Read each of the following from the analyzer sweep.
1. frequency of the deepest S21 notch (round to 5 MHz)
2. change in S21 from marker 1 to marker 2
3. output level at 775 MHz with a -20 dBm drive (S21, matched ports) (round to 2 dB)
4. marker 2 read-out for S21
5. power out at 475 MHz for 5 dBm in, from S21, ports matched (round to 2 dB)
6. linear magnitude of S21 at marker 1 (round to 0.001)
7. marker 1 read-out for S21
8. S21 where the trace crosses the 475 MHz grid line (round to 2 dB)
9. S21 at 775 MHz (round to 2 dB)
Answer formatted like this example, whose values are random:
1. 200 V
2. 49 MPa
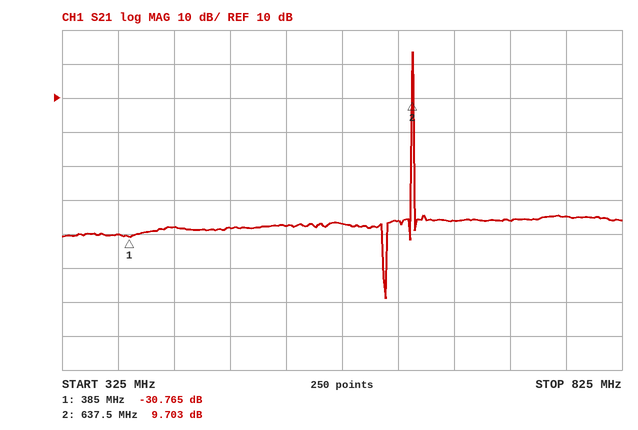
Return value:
1. 615 MHz
2. 40.468 dB
3. -44 dBm
4. 9.703 dB
5. -24 dBm
6. 0.029
7. -30.765 dB
8. -28 dB
9. -24 dB
